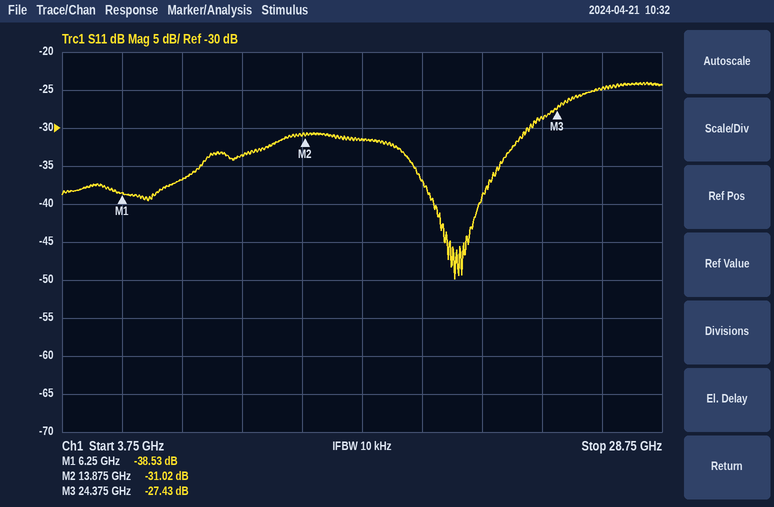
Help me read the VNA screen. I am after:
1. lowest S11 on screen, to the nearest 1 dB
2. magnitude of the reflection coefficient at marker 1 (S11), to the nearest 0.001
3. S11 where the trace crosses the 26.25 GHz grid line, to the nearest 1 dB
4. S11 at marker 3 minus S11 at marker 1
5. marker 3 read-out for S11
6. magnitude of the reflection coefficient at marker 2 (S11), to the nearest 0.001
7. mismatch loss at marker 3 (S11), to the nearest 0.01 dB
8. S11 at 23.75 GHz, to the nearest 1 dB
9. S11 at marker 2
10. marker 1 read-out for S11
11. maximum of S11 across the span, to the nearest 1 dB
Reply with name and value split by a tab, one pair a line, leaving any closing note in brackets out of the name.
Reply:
lowest S11 on screen, to the nearest 1 dB	-50 dB
magnitude of the reflection coefficient at marker 1 (S11), to the nearest 0.001	0.012
S11 where the trace crosses the 26.25 GHz grid line, to the nearest 1 dB	-25 dB
S11 at marker 3 minus S11 at marker 1	11.10 dB
marker 3 read-out for S11	-27.43 dB
magnitude of the reflection coefficient at marker 2 (S11), to the nearest 0.001	0.028
mismatch loss at marker 3 (S11), to the nearest 0.01 dB	0.01 dB
S11 at 23.75 GHz, to the nearest 1 dB	-29 dB
S11 at marker 2	-31.02 dB
marker 1 read-out for S11	-38.53 dB
maximum of S11 across the span, to the nearest 1 dB	-24 dB
